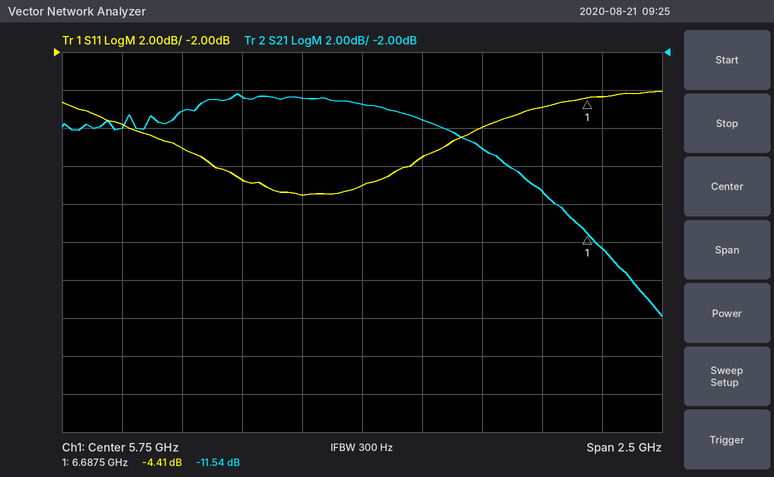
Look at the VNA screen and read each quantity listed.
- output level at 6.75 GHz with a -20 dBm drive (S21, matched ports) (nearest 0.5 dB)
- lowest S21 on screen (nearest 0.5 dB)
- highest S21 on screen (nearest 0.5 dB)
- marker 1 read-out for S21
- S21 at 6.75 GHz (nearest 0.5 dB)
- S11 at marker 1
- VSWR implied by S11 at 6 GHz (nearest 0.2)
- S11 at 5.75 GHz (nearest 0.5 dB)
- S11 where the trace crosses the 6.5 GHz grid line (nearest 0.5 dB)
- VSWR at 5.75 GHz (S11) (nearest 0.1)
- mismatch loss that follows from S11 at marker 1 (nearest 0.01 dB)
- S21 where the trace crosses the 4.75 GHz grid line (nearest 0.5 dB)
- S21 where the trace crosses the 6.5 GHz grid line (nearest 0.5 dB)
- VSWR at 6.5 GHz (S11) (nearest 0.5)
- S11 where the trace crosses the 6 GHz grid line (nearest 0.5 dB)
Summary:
-32.5 dBm
-16.0 dB
-4.0 dB
-11.54 dB
-12.5 dB
-4.41 dB
2.4
-9.0 dB
-5.0 dB
2.1
1.95 dB
-6.0 dB
-9.5 dB
3.5
-7.5 dB
